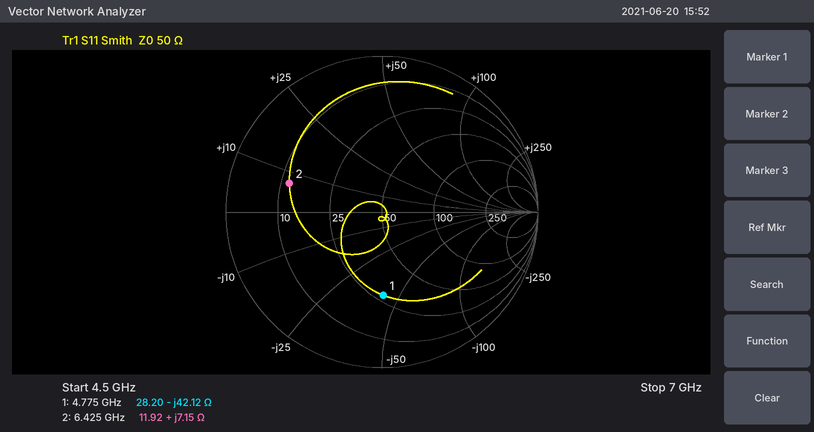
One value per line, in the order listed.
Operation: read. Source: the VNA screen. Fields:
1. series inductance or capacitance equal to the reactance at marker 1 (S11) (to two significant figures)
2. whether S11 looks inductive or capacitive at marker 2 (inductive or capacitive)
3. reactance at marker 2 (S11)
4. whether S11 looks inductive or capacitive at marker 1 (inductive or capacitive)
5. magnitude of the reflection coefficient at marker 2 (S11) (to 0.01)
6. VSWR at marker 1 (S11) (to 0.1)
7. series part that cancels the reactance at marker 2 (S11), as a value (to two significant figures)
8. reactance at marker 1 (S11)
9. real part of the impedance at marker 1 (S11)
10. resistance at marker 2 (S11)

790 fF
inductive
+7.15 Ω
capacitive
0.62
3.3
3.5 pF
-42.12 Ω
28.20 Ω
11.92 Ω
